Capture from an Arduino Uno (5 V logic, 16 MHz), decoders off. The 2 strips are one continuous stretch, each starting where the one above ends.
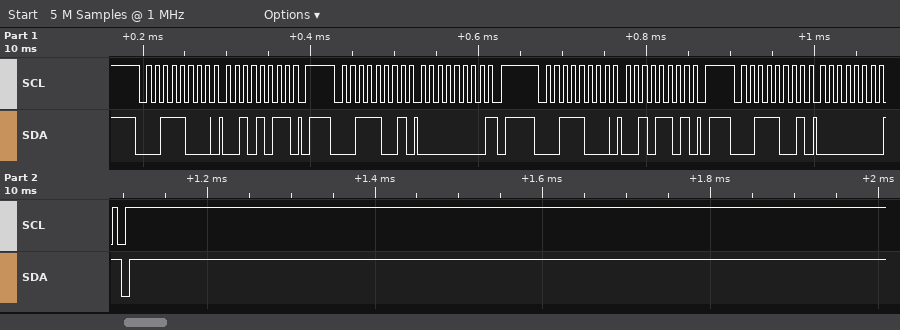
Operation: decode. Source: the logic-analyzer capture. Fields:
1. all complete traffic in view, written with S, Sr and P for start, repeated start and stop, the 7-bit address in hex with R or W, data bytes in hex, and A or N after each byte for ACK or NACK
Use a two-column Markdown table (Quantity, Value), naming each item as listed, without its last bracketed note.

| Quantity | Value |
|---|---|
| all complete traffic in view, written with S, Sr and P for start, repeated start and stop, the 7-bit address in hex with R or W, data bytes in hex, and A or N after each byte for ACK or NACK | S 1CW A 2B A P S 1CR A 00 N P S 1CW A 2D A P S 1CR A 00 N P |
